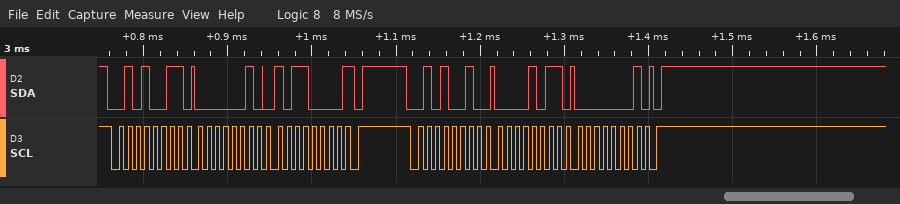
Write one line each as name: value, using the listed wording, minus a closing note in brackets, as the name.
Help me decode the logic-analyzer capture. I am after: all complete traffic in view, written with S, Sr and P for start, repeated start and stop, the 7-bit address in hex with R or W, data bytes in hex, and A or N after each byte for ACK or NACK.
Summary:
all complete traffic in view, written with S, Sr and P for start, repeated start and stop, the 7-bit address in hex with R or W, data bytes in hex, and A or N after each byte for ACK or NACK: S 29R A 02 A B0 N P S 29W A 0B A 01 A P
